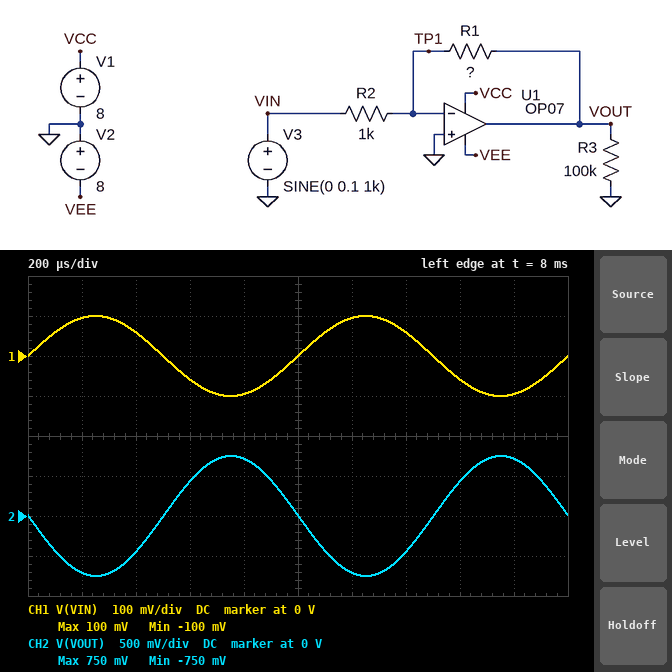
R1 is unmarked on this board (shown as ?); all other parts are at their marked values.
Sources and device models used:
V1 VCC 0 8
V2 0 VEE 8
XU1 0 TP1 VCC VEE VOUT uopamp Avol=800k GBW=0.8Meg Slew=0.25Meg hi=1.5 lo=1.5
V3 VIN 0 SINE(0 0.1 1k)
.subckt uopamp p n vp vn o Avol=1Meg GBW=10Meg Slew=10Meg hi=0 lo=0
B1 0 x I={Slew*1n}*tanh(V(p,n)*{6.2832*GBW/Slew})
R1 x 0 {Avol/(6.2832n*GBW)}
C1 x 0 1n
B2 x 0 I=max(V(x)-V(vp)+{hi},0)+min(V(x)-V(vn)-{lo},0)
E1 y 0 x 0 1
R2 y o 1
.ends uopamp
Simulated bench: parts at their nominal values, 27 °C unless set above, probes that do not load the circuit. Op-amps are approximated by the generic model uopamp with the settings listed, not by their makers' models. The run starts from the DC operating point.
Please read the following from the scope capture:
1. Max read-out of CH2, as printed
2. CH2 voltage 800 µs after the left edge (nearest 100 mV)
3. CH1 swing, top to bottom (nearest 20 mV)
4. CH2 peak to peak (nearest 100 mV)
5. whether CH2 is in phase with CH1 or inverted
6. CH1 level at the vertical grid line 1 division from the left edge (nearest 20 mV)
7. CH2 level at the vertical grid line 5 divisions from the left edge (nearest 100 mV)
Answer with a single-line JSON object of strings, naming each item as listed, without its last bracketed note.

{"Max read-out of CH2, as printed": "750 mV", "CH2 voltage 800 µs after the left edge": "700 mV", "CH1 swing, top to bottom": "200 mV", "CH2 peak to peak": "1.5 V", "whether CH2 is in phase with CH1 or inverted": "inverted", "CH1 level at the vertical grid line 1 division from the left edge": "100 mV", "CH2 level at the vertical grid line 5 divisions from the left edge": "0 V"}
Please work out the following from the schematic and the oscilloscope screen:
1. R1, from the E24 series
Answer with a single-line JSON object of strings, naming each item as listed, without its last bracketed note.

{"R1, from the E24 series": "7.5 kΩ"}
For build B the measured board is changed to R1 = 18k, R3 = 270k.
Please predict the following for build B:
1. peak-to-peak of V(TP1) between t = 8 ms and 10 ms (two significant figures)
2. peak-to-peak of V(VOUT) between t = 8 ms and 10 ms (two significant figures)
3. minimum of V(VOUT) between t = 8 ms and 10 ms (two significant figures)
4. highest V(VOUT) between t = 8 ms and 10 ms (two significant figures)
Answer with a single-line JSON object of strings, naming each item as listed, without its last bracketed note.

{"peak-to-peak of V(TP1) between t = 8 ms and 10 ms": "4.5 mV", "peak-to-peak of V(VOUT) between t = 8 ms and 10 ms": "3.6 V", "minimum of V(VOUT) between t = 8 ms and 10 ms": "-1.8 V", "highest V(VOUT) between t = 8 ms and 10 ms": "1.8 V"}
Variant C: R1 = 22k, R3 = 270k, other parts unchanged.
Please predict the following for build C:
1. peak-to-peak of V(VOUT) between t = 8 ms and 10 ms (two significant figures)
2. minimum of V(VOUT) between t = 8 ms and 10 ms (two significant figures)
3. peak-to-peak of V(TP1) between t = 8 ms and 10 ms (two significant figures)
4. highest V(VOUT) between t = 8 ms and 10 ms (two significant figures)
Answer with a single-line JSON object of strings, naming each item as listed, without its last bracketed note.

{"peak-to-peak of V(VOUT) between t = 8 ms and 10 ms": "4.4 V", "minimum of V(VOUT) between t = 8 ms and 10 ms": "-2.2 V", "peak-to-peak of V(TP1) between t = 8 ms and 10 ms": "5.5 mV", "highest V(VOUT) between t = 8 ms and 10 ms": "2.2 V"}
